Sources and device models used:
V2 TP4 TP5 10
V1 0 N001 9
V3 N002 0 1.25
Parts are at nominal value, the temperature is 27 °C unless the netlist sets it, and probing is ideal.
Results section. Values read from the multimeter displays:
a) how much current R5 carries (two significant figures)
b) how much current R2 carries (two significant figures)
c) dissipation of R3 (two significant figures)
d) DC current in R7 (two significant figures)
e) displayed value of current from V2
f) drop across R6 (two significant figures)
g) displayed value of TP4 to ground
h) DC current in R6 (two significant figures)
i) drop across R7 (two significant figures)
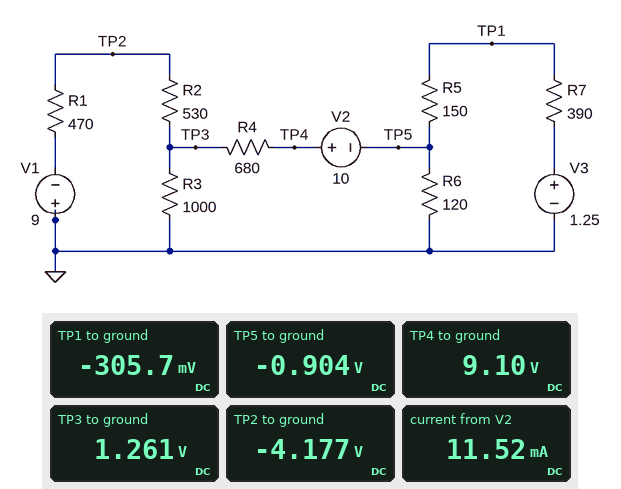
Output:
4.0 mA
10 mA
1.6 mW
4.0 mA
11.52 mA
900 mV
9.10 V
7.5 mA
1.6 V
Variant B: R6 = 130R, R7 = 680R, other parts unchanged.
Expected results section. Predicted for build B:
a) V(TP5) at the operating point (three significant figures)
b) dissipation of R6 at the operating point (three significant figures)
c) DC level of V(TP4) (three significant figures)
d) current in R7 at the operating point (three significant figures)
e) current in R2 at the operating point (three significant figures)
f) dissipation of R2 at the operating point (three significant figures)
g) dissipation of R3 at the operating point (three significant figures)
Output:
-1.11 V
9.42 mW
8.89 V
2.84 mA
10.2 mA
54.9 mW
1.38 mW
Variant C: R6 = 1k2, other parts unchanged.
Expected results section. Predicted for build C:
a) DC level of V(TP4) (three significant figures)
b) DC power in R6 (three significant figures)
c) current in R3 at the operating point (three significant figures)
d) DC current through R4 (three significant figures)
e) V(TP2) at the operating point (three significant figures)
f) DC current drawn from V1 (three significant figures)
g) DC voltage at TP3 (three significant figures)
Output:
7.18 V
6.64 mW
448 µA
9.90 mA
-4.56 V
9.45 mA
448 mV
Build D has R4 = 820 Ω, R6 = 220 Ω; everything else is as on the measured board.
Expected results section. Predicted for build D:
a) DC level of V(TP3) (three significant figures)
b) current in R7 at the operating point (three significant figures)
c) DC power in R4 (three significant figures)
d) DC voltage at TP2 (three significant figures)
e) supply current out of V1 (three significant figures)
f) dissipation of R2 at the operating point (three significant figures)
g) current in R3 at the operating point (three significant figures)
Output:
533 mV
4.56 mA
83.1 mW
-4.52 V
9.53 mA
48.2 mW
533 µA
